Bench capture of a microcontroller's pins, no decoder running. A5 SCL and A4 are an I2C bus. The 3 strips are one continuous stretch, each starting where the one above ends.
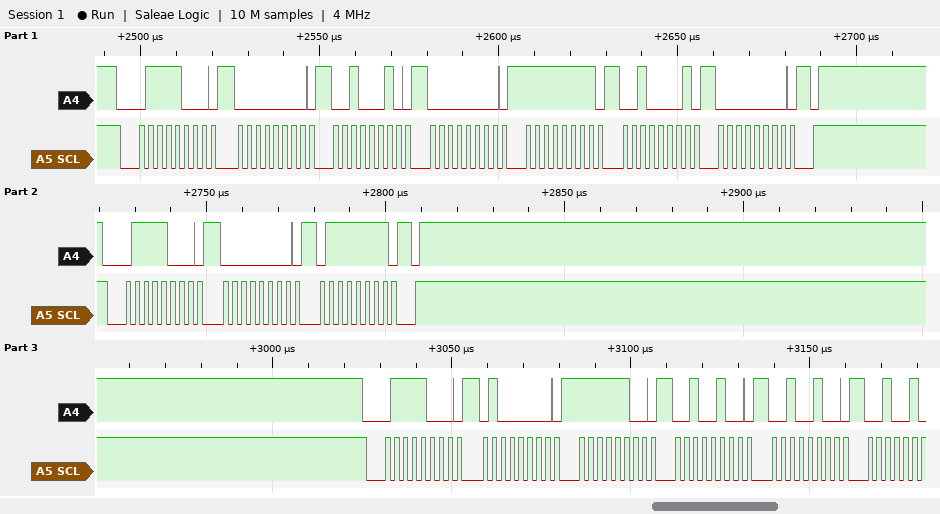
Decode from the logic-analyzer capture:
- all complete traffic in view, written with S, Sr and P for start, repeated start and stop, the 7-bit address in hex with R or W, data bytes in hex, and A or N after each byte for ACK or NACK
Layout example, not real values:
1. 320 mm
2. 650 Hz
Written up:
1. S 3CW A 00 A 22 A 00 A FF A 21 A 00 A P S 3CW A 00 A 7F A P S 3CW A 40 A FC A 24 A 24 A
